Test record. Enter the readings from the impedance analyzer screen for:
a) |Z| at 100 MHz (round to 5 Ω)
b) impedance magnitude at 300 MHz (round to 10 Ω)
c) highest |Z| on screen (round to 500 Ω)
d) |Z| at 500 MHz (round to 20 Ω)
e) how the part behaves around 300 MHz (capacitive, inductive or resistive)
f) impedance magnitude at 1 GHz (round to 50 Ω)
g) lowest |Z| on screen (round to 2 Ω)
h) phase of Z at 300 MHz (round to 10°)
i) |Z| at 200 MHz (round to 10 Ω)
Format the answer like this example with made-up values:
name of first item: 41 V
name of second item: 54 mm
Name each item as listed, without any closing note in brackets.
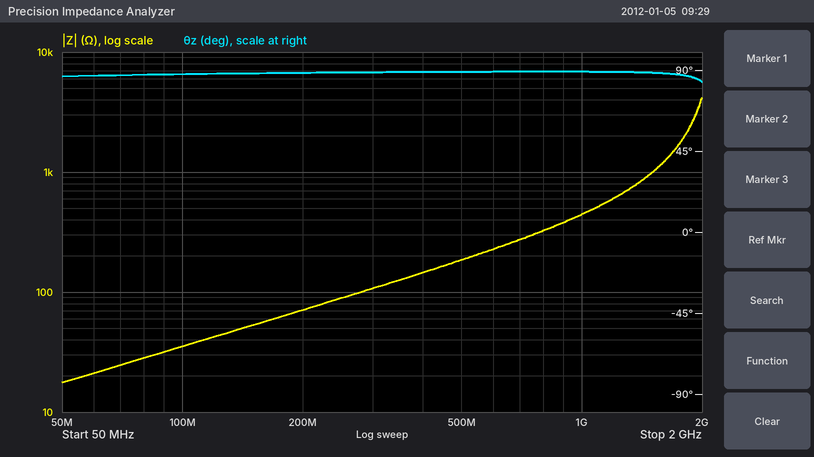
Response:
|Z| at 100 MHz: 35 Ω
impedance magnitude at 300 MHz: 110 Ω
highest |Z| on screen: 4.0 kΩ
|Z| at 500 MHz: 180 Ω
how the part behaves around 300 MHz: inductive
impedance magnitude at 1 GHz: 450 Ω
lowest |Z| on screen: 18 Ω
phase of Z at 300 MHz: 90°
|Z| at 200 MHz: 70 Ω
